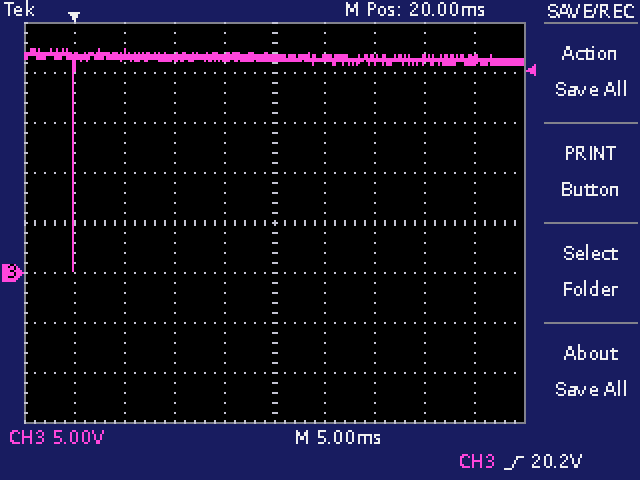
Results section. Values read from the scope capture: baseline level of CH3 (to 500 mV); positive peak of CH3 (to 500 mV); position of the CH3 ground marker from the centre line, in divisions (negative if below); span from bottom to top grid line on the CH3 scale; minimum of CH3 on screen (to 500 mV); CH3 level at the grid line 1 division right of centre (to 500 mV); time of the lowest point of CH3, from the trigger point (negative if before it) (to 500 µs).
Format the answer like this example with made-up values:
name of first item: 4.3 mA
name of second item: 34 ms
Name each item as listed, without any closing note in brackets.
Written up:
baseline level of CH3: 21.5 V
positive peak of CH3: 22.5 V
position of the CH3 ground marker from the centre line, in divisions: -1.0 div
span from bottom to top grid line on the CH3 scale: 40 V
minimum of CH3 on screen: 0.0 V
CH3 level at the grid line 1 division right of centre: 21.5 V
time of the lowest point of CH3, from the trigger point (negative if before it): 0.0 ms
